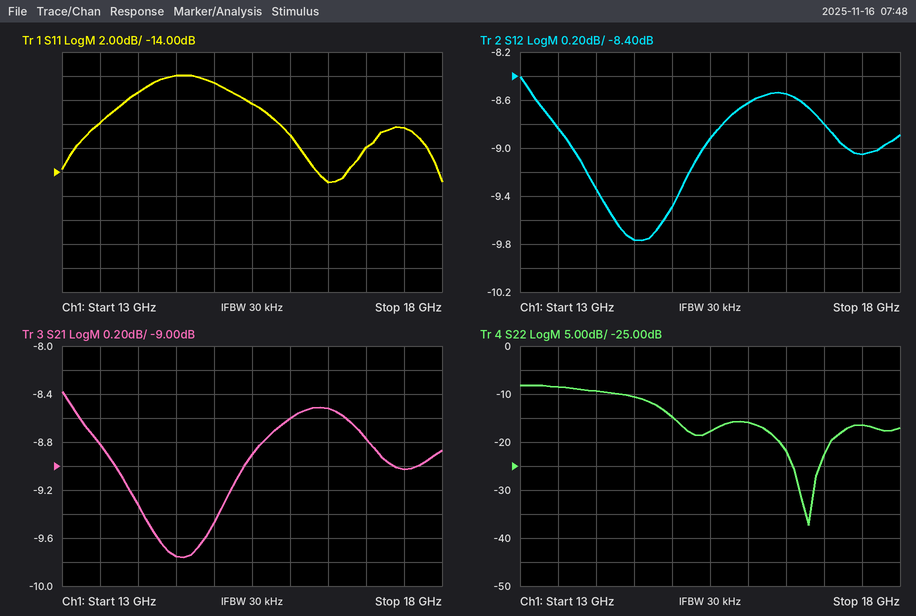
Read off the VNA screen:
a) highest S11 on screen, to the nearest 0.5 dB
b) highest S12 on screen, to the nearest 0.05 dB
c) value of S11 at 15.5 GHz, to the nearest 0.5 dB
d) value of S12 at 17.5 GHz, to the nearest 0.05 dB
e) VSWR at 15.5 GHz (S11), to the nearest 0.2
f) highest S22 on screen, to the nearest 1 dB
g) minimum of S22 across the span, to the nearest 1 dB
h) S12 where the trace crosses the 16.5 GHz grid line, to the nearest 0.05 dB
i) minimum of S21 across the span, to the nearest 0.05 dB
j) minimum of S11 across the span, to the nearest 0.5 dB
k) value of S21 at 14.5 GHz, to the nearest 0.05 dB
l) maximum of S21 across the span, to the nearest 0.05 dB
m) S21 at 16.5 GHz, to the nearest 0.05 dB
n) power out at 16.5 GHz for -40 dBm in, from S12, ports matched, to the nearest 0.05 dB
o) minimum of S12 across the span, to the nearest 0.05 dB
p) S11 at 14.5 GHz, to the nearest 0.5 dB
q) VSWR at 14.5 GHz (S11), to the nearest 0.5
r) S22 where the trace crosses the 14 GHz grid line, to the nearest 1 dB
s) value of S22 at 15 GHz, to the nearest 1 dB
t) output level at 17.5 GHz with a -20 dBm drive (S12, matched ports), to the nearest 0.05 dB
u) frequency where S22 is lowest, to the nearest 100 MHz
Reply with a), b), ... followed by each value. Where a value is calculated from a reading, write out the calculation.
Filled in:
a) -6.0 dB
b) -8.40 dB
c) -8.5 dB
d) -9.05 dB
e) |Γ| = 10^(-8.5/20) = 0.3758; VSWR = (1 + 0.3758)/(1 − 0.3758) ≈ 2.2
f) -8 dB
g) -37 dB
h) -8.55 dB
i) -9.75 dB
j) -15.0 dB
k) -9.75 dB
l) -8.40 dB
m) -8.50 dB
n) -40 dBm + (-8.55 dB) = -48.55 dBm
o) -9.75 dB
p) -6.0 dB
q) |Γ| = 10^(-6/20) = 0.5012; VSWR = (1 + 0.5012)/(1 − 0.5012) ≈ 3.0
r) -9 dB
s) -15 dB
t) -20 dBm + (-9.05 dB) = -29.05 dBm
u) 16.8 GHz
